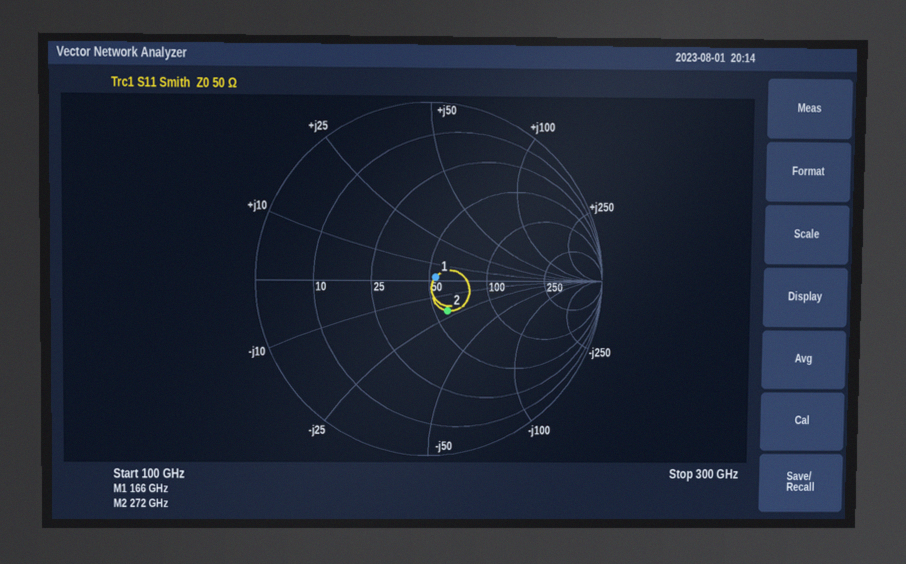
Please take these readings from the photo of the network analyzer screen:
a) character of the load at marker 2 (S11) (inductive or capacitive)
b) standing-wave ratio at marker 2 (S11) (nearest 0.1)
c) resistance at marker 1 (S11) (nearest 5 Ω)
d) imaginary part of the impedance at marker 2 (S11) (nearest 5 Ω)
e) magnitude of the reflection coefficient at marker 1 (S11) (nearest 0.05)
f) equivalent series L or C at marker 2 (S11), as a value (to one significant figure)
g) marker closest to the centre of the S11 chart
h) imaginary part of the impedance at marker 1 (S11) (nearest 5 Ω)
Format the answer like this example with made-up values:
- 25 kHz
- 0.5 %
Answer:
- capacitive
- 1.5
- 55 Ω
- -20 Ω
- 0.05
- 30 fF
- marker 1
- 0 Ω
